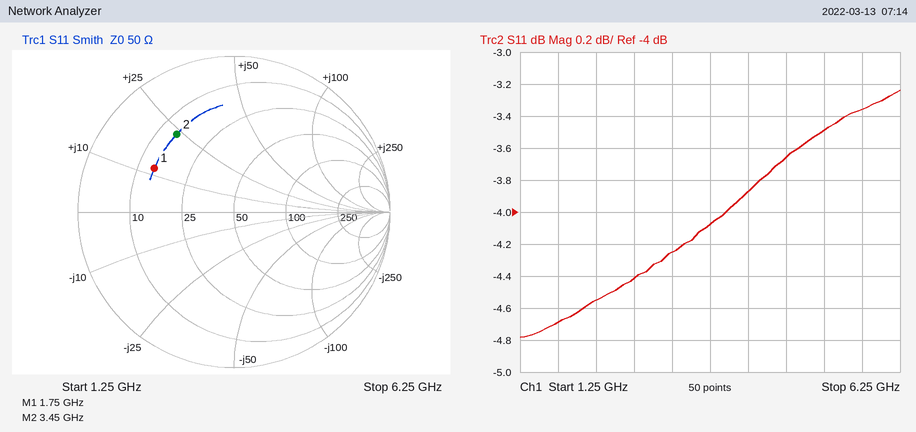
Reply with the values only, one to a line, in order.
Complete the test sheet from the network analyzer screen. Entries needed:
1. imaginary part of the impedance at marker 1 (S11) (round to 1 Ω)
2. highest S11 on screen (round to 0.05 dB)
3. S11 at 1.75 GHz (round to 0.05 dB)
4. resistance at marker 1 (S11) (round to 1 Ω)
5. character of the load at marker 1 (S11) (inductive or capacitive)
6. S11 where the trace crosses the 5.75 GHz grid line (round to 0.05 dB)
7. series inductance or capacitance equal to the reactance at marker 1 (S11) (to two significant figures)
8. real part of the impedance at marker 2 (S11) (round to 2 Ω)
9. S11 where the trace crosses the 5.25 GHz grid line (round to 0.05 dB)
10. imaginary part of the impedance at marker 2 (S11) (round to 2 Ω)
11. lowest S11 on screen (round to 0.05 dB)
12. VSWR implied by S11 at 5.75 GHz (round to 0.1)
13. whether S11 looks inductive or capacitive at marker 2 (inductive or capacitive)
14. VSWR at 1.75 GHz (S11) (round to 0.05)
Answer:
+12 Ω
-3.25 dB
-4.70 dB
14 Ω
inductive
-3.35 dB
1.1 nH
14 Ω
-3.50 dB
+24 Ω
-4.80 dB
5.2
inductive
3.80
